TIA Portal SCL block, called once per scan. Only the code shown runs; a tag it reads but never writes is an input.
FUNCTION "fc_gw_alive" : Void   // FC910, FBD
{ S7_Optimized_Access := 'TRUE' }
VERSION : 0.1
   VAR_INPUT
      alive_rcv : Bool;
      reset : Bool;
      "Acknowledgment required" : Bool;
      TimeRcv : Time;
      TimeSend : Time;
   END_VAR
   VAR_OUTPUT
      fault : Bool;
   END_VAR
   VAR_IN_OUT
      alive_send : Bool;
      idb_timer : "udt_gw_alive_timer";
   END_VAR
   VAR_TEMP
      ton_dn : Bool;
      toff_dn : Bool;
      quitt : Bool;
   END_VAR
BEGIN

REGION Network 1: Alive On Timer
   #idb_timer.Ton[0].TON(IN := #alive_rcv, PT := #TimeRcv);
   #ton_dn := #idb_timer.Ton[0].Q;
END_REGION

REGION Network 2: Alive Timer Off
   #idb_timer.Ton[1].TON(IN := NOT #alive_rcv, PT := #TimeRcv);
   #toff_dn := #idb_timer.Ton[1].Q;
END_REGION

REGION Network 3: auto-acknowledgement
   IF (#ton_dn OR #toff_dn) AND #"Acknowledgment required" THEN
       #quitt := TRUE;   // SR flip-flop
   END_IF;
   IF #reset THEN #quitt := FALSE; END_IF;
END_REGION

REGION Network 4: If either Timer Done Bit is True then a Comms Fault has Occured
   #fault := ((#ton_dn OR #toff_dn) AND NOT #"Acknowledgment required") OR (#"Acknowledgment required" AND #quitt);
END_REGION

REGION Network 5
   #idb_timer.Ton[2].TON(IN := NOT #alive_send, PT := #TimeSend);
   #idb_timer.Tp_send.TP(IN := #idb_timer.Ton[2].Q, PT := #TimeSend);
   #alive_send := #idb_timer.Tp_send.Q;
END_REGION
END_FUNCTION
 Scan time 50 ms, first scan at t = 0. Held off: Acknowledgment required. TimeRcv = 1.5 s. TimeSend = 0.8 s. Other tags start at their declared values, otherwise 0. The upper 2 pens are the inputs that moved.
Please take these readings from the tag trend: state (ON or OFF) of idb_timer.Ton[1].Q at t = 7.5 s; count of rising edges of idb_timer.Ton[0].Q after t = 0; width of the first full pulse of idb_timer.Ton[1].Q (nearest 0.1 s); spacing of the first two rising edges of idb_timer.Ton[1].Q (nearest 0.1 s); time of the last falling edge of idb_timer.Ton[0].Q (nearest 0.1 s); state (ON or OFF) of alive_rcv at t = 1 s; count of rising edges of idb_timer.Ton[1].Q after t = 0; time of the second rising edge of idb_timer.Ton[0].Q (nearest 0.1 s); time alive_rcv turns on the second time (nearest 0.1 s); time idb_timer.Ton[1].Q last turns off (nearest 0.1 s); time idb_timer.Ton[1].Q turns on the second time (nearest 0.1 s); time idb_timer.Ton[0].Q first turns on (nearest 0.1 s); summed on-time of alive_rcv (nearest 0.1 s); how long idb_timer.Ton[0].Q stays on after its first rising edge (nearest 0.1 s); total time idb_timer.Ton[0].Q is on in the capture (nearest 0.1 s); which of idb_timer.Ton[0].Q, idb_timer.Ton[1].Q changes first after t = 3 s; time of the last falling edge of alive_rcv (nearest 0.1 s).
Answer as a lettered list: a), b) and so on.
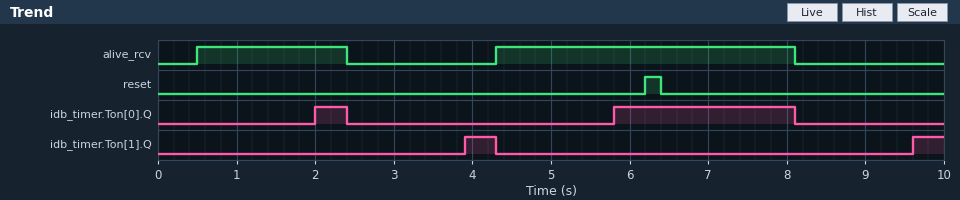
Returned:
a) OFF
b) 2
c) 0.4 s
d) 5.7 s
e) 8.1 s
f) ON
g) 2
h) 5.8 s
i) 4.3 s
j) 4.3 s
k) 9.6 s
l) 2.0 s
m) 5.7 s
n) 0.4 s
o) 2.7 s
p) idb_timer.Ton[1].Q
q) 8.1 s
